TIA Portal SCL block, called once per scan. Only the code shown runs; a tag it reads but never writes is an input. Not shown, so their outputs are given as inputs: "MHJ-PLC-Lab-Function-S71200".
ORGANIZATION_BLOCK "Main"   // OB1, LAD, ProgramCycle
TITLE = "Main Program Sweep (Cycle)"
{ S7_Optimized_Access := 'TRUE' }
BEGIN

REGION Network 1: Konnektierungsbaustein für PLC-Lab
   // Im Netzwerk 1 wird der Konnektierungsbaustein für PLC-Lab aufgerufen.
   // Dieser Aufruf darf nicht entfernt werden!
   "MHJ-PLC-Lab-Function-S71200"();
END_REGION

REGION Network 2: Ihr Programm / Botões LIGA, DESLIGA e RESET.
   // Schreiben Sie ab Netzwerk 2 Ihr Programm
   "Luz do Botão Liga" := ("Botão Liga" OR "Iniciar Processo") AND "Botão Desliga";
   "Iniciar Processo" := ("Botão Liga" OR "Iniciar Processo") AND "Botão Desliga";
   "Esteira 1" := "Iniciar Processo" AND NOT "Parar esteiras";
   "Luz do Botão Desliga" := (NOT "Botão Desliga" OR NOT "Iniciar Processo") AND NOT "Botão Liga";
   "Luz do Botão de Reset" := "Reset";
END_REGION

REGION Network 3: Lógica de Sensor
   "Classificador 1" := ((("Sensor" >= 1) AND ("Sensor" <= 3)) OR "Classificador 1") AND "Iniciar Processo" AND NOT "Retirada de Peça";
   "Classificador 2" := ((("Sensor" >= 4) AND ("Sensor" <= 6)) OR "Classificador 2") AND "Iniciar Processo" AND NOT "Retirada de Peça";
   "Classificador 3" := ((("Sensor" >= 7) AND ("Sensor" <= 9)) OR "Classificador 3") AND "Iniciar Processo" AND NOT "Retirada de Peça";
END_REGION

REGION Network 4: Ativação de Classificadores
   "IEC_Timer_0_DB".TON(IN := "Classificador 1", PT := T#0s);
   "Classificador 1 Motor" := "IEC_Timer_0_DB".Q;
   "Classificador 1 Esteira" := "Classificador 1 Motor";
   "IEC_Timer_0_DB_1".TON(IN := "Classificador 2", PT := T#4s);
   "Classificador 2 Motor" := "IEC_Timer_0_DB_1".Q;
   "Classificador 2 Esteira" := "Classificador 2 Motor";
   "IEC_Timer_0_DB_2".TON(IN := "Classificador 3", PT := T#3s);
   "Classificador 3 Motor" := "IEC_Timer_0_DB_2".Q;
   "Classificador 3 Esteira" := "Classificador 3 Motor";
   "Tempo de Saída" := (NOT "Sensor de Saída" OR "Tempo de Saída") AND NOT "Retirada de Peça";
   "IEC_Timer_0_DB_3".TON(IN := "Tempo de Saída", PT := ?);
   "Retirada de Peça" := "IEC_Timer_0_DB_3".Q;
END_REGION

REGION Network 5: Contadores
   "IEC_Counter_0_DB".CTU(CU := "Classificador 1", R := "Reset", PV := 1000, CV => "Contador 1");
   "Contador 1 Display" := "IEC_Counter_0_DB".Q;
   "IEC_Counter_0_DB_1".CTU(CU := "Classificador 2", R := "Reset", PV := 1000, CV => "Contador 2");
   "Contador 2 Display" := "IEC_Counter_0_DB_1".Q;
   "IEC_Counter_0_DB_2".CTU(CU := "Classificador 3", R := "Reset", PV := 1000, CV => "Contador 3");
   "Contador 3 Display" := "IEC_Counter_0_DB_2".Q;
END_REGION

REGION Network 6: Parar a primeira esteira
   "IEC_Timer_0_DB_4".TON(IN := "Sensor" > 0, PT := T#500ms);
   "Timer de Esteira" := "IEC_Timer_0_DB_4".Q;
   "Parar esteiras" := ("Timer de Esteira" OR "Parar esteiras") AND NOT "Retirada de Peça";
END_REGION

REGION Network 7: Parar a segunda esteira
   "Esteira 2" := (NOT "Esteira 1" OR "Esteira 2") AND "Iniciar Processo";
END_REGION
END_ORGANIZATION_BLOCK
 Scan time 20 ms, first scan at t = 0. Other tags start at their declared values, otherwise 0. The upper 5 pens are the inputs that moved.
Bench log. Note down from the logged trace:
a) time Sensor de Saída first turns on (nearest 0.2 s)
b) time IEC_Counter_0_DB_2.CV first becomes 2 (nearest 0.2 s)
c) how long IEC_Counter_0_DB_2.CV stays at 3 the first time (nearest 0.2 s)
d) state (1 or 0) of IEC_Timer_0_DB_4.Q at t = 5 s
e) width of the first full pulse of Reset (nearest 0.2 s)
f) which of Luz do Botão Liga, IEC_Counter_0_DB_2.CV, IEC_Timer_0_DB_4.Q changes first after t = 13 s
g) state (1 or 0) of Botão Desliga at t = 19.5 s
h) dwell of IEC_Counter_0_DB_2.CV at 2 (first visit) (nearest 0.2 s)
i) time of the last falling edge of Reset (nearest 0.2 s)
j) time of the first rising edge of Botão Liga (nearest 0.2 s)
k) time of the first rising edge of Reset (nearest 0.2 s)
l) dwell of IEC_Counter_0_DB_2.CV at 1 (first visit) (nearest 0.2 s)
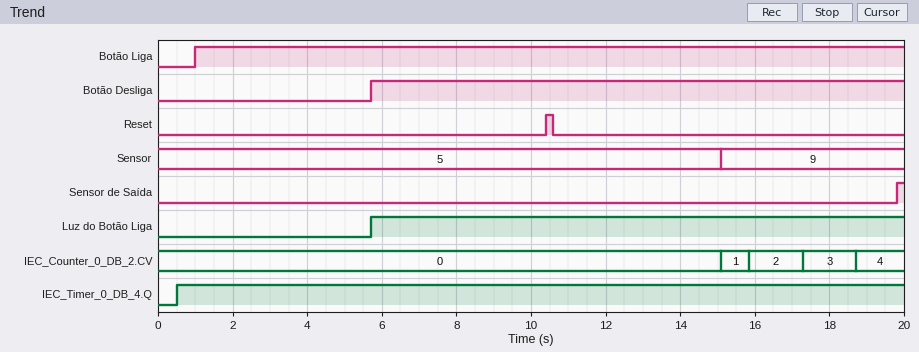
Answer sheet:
19.8 s
15.8 s
1.4 s
1
0.2 s
IEC_Counter_0_DB_2.CV
1
1.4 s
10.6 s
1.0 s
10.4 s
0.8 s
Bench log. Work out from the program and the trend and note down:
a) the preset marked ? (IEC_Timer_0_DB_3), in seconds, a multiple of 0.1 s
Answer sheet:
1.4 s
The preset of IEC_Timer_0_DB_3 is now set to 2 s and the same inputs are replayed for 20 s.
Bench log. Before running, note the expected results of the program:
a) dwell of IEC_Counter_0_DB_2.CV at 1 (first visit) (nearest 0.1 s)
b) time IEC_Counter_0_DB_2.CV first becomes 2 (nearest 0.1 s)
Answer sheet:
1.2 s
16.3 s
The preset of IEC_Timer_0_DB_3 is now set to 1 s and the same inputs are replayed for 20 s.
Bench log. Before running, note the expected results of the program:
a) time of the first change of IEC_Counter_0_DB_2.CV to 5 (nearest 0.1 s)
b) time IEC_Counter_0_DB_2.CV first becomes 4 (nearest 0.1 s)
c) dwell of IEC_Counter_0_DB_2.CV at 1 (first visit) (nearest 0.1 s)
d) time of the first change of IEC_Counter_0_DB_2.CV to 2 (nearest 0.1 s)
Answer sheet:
18.7 s
17.7 s
0.5 s
15.6 s
